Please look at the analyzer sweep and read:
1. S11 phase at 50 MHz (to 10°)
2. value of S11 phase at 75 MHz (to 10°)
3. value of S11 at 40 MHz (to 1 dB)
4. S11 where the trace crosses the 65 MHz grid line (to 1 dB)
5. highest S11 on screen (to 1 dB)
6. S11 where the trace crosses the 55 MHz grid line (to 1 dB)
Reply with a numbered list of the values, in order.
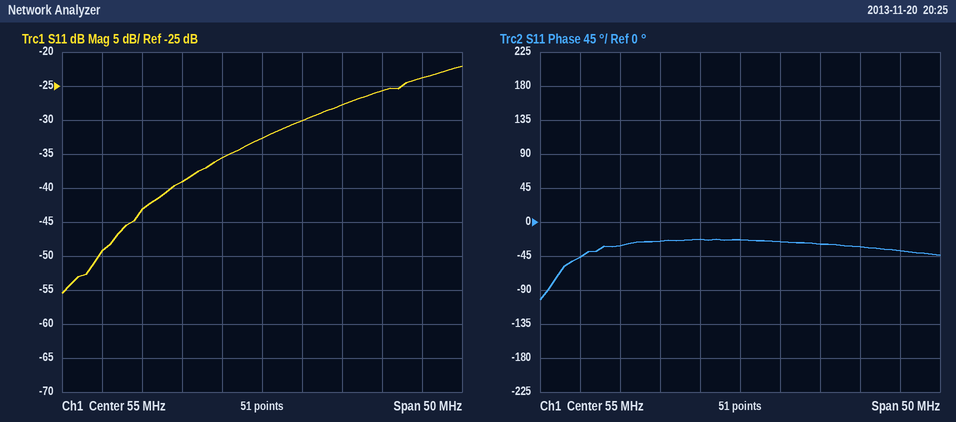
1. -20°
2. -40°
3. -43 dB
4. -28 dB
5. -22 dB
6. -33 dB
